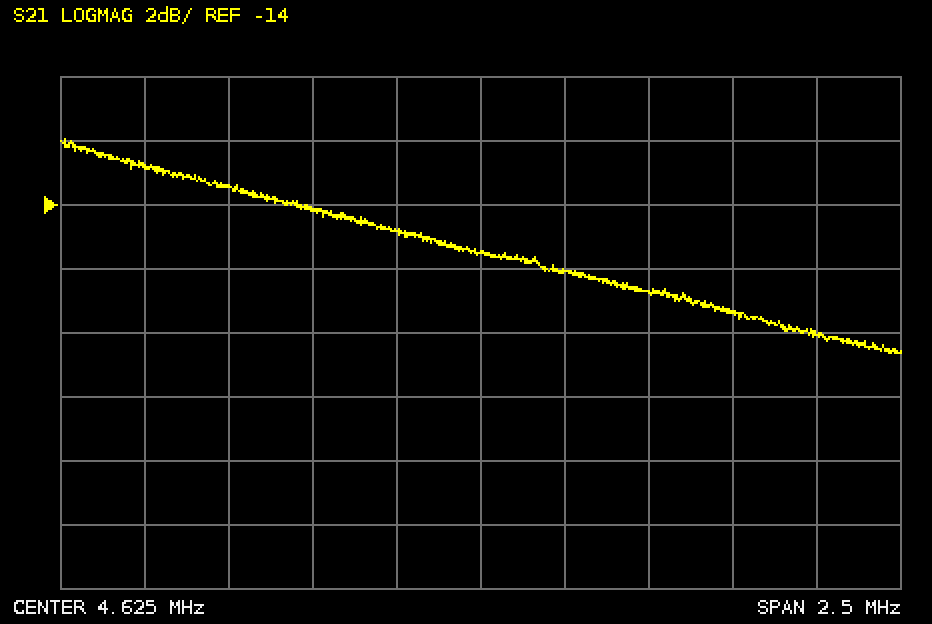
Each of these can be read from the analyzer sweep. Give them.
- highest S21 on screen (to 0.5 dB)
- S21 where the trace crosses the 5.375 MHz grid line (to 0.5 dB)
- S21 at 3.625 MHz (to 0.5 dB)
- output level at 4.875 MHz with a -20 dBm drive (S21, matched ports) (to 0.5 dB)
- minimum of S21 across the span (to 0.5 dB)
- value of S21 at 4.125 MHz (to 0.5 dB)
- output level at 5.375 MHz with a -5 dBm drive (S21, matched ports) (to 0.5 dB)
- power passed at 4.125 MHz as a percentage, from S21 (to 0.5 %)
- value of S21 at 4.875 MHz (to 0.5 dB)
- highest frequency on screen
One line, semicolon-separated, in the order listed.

-12.0 dB; -17.5 dB; -13.0 dB; -36.0 dBm; -18.5 dB; -14.0 dB; -22.5 dBm; 4.0 %; -16.0 dB; 5.875 MHz
